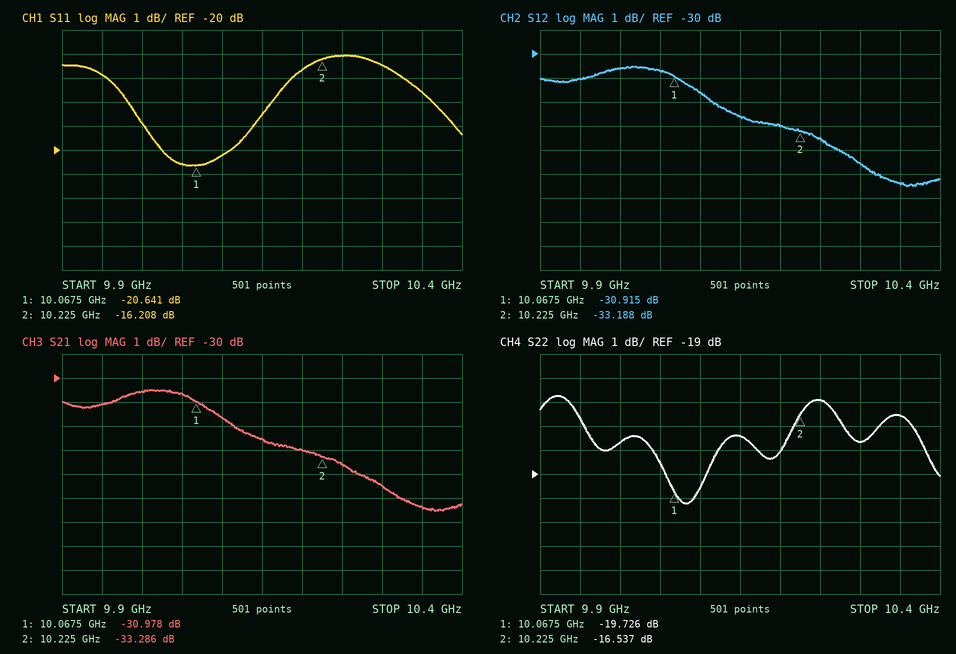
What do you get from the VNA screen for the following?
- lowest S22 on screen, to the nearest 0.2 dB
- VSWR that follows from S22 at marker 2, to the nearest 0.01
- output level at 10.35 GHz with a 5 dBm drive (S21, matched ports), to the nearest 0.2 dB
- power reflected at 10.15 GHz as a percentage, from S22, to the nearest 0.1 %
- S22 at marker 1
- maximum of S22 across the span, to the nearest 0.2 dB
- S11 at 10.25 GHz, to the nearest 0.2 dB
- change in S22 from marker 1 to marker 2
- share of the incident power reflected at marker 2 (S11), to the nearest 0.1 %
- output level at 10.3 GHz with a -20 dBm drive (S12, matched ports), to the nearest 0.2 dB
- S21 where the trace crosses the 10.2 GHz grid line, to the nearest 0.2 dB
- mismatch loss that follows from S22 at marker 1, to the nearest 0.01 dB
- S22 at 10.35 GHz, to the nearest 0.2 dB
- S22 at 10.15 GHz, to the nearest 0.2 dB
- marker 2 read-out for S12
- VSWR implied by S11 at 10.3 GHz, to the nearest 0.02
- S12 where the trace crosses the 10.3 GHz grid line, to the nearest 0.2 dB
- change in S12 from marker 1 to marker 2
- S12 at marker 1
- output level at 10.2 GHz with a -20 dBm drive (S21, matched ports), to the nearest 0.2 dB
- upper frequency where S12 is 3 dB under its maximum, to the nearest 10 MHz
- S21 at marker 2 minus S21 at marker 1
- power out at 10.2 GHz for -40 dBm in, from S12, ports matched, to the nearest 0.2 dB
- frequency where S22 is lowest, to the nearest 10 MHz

-20.2 dB
1.35
-30.4 dBm
1.8 %
-19.726 dB
-15.8 dB
-16.0 dB
3.189 dB
2.4 %
-54.6 dBm
-33.0 dB
0.05 dB
-16.6 dB
-17.4 dB
-33.188 dB
1.36
-34.6 dB
-2.273 dB
-30.915 dB
-53.0 dBm
10.25 GHz
-2.308 dB
-73.0 dBm
10.08 GHz
